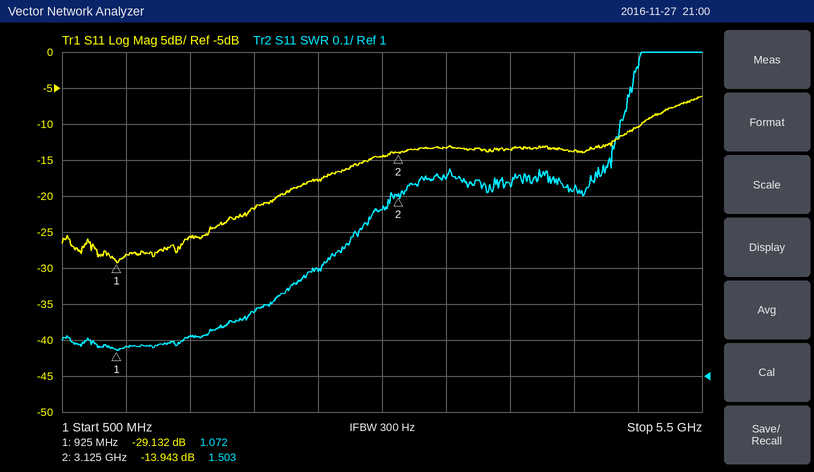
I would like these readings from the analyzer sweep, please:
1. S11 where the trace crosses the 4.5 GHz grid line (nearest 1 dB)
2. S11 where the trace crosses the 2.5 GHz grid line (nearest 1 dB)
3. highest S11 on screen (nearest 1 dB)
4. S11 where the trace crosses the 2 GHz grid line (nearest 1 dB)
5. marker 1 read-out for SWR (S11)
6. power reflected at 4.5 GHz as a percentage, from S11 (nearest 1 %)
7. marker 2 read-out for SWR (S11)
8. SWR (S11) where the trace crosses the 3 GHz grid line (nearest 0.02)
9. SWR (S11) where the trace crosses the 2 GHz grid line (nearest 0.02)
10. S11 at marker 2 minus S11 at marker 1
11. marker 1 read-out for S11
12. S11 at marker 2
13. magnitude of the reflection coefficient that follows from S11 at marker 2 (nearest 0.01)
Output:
-14 dB
-18 dB
-6 dB
-22 dB
1.072
4 %
1.503
1.46
1.18
15.189 dB
-29.132 dB
-13.943 dB
0.20
